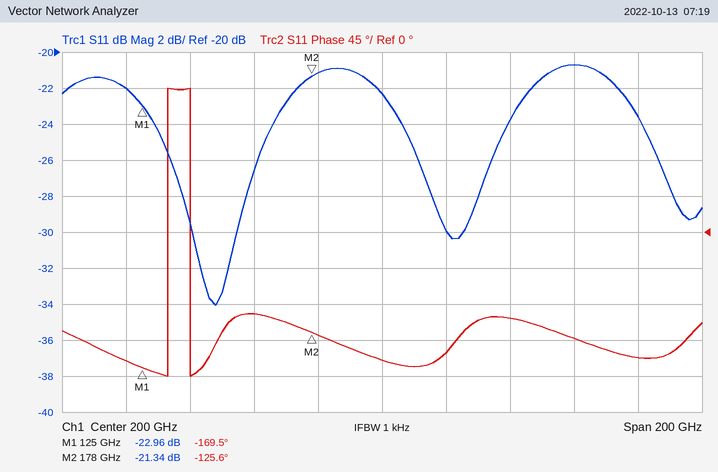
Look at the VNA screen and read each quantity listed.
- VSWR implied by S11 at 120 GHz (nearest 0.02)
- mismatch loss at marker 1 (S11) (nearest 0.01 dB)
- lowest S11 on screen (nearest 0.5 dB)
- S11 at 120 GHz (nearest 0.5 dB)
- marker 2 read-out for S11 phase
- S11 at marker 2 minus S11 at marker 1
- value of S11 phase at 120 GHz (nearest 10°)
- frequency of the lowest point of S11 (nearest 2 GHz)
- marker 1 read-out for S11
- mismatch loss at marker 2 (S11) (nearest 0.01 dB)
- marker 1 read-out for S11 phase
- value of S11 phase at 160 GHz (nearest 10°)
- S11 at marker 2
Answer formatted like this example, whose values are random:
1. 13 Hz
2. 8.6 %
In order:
1. 1.18
2. 0.02 dB
3. -34.0 dB
4. -22.0 dB
5. -125.6°
6. 1.62 dB
7. -160°
8. 148 GHz
9. -22.96 dB
10. 0.03 dB
11. -169.5°
12. -100°
13. -21.34 dB
